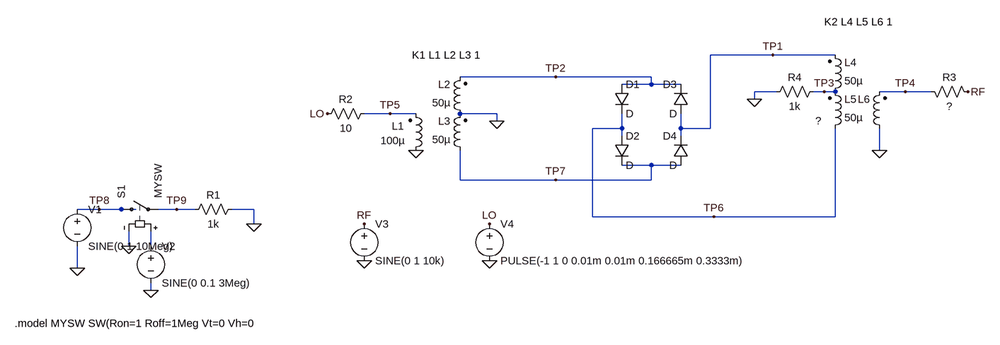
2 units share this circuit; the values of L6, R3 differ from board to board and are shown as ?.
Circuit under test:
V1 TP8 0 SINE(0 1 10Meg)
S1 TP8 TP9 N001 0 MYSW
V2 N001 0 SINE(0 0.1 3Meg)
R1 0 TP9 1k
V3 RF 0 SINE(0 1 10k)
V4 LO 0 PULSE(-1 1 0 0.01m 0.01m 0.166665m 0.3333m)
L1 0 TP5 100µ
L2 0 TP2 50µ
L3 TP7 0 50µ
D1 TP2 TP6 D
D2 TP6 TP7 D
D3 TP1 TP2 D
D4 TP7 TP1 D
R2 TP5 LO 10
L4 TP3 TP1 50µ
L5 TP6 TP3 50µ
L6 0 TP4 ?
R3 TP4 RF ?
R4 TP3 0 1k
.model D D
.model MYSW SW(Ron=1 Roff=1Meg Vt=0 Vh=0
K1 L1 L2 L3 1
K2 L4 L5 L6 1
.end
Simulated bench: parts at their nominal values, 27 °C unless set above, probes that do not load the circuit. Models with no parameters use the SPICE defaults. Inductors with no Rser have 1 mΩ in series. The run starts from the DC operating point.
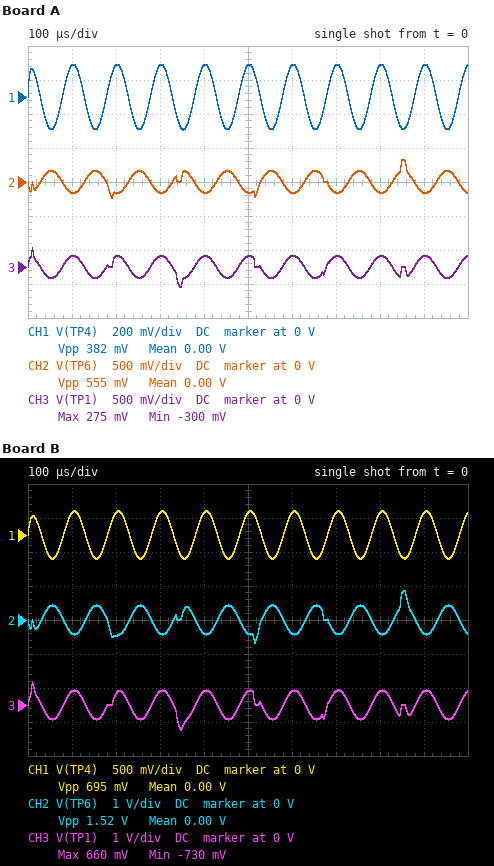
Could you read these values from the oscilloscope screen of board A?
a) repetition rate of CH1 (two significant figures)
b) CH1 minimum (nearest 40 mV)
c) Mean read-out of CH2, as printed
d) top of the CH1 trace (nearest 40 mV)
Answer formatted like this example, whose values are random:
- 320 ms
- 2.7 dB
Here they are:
- 10 kHz
- -200 mV
- 0.00 V
- 200 mV
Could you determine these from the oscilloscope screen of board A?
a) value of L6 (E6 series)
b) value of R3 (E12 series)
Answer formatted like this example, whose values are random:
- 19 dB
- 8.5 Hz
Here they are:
- 68 µH
- 22 Ω
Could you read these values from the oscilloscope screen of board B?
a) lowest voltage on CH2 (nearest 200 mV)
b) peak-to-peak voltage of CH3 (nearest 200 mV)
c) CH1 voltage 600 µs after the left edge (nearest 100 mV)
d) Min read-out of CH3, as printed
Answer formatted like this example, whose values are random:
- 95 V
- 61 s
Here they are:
- -600 mV
- 1.4 V
- 300 mV
- -730 mV
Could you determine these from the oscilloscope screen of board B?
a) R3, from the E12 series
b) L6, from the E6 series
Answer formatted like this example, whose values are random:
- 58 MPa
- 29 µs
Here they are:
- 5.6 Ω
- 33 µH
